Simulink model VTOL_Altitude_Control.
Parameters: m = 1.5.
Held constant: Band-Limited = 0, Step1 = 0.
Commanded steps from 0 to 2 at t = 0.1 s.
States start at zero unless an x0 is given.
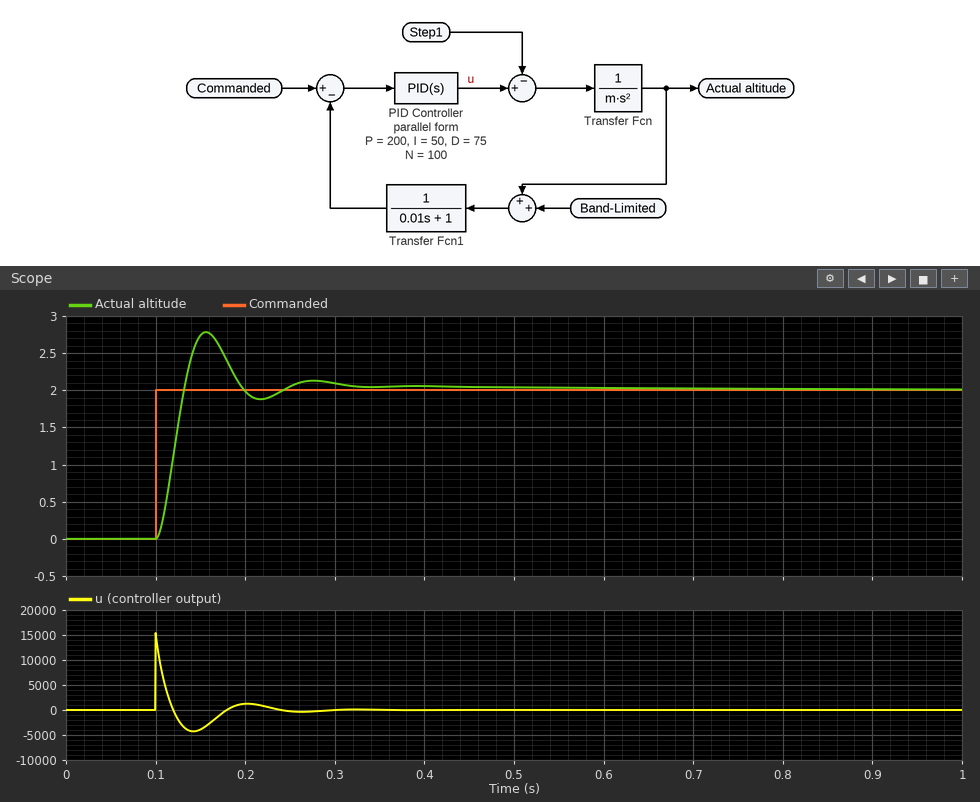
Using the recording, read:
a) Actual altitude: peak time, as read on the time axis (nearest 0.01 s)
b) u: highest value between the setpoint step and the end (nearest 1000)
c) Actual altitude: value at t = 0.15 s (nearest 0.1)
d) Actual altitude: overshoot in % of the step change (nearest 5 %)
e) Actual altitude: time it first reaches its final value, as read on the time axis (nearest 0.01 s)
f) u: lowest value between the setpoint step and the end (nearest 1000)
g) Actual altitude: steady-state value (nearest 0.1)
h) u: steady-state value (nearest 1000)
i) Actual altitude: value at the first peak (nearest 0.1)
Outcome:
0.16 s
15000
2.7
40 %
0.13 s
-4000
2.0
0
2.8
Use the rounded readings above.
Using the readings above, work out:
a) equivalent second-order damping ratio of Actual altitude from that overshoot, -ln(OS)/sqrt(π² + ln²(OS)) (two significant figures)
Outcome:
0.28
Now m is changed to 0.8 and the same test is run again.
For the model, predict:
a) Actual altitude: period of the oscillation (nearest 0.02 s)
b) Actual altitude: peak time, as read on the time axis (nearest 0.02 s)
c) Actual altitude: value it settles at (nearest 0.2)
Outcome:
0.08 s
0.14 s
2.0
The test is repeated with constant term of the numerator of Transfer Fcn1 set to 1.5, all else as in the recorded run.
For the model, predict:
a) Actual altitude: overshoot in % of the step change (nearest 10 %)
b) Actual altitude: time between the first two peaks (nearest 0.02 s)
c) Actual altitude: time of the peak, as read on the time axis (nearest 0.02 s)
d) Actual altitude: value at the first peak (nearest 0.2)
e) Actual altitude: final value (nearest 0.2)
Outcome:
60 %
0.10 s
0.14 s
2.2
1.4
